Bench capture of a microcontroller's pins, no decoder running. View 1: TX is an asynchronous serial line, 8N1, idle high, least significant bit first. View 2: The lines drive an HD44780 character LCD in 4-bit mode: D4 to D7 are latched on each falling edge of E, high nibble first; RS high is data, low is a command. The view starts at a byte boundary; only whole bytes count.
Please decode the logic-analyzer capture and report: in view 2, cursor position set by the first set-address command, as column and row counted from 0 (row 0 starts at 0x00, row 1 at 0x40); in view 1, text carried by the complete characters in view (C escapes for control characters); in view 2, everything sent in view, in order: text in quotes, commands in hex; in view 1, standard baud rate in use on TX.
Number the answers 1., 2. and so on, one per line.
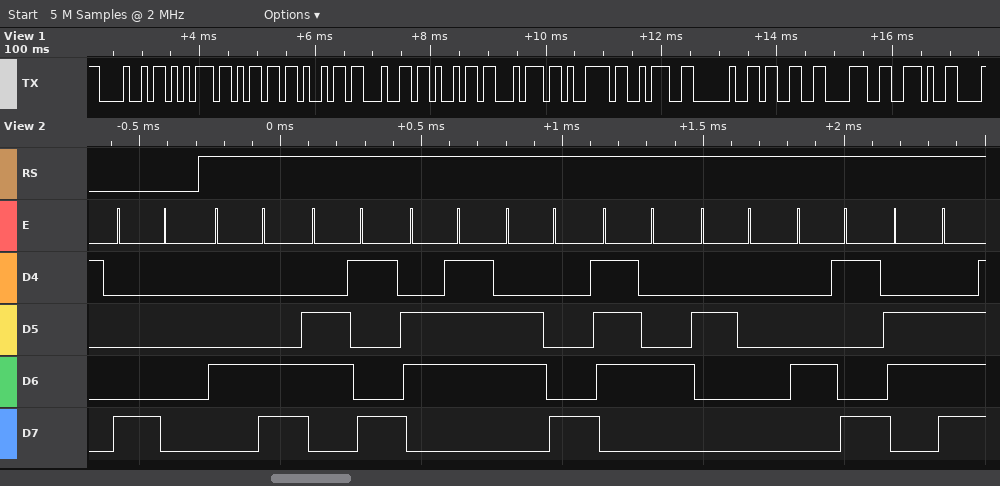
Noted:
1. column 0, row 0
2. "Humidity: 38."
3. 0x80 "Light In"
4. 9600 baud
